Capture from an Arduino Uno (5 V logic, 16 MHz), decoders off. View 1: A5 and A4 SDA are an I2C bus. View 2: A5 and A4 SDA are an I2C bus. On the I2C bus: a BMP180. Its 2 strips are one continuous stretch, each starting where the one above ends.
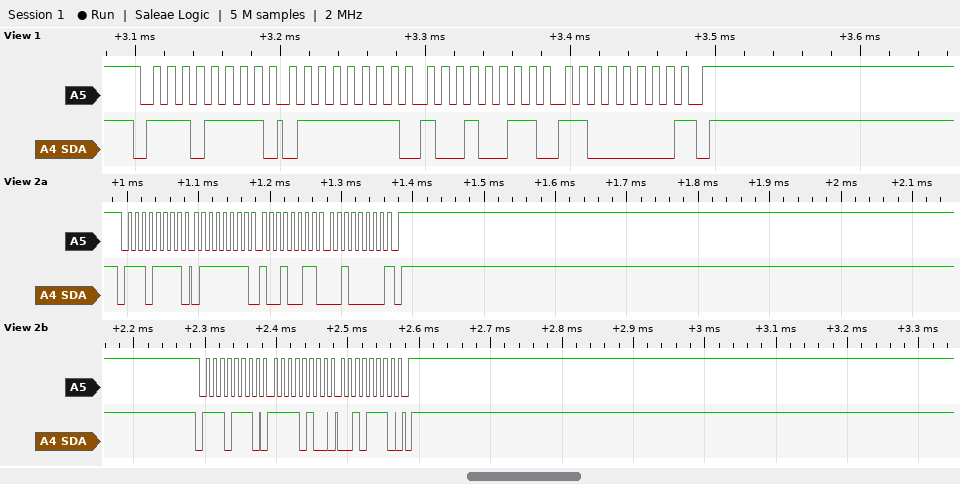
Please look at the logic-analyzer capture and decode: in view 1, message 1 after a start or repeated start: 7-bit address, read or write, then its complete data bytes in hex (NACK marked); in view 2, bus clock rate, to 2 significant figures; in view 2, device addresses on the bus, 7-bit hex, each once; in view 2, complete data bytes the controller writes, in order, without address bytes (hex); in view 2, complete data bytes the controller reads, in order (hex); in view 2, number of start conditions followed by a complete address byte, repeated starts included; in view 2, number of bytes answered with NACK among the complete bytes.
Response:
0x77 read: 7F 93 C0 NACK
100 kHz
0x77
F4 2E
7F 93 20
2
1
